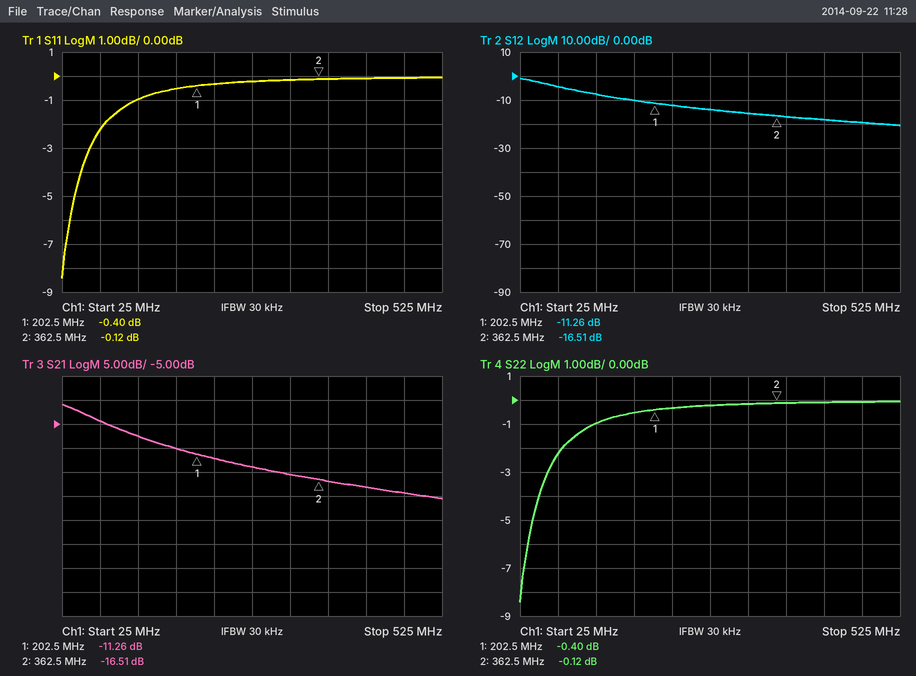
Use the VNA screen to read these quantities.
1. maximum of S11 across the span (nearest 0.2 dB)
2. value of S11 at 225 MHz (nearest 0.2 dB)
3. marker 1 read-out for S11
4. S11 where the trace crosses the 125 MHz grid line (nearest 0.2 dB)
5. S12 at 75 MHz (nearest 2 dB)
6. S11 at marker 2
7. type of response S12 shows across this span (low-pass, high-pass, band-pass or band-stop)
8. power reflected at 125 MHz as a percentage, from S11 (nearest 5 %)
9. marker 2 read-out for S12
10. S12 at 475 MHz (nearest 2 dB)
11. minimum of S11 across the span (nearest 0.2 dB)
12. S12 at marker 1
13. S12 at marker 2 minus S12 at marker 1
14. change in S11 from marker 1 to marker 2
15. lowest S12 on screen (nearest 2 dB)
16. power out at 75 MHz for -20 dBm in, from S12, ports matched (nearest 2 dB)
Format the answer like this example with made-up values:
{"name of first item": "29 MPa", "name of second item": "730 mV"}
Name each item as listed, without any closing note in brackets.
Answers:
{"maximum of S11 across the span": "0.0 dB", "value of S11 at 225 MHz": "-0.4 dB", "marker 1 read-out for S11": "-0.40 dB", "S11 where the trace crosses the 125 MHz grid line": "-1.0 dB", "S12 at 75 MHz": "-4 dB", "S11 at marker 2": "-0.12 dB", "type of response S12 shows across this span": "low-pass", "power reflected at 125 MHz as a percentage, from S11": "80 %", "marker 2 read-out for S12": "-16.51 dB", "S12 at 475 MHz": "-20 dB", "minimum of S11 across the span": "-8.4 dB", "S12 at marker 1": "-11.26 dB", "S12 at marker 2 minus S12 at marker 1": "-5.25 dB", "change in S11 from marker 1 to marker 2": "0.28 dB", "lowest S12 on screen": "-20 dB", "power out at 75 MHz for -20 dBm in, from S12, ports matched": "-24 dBm"}
